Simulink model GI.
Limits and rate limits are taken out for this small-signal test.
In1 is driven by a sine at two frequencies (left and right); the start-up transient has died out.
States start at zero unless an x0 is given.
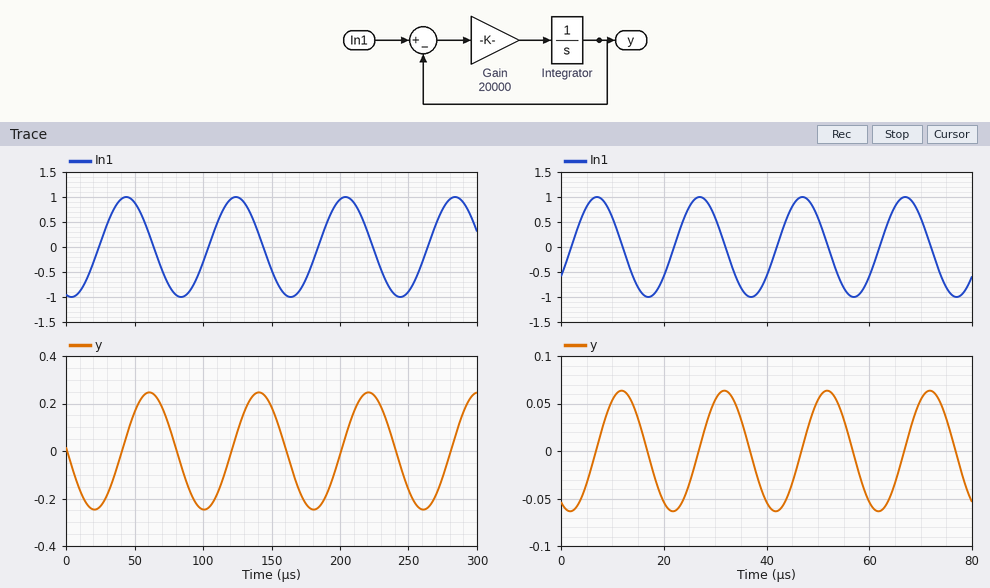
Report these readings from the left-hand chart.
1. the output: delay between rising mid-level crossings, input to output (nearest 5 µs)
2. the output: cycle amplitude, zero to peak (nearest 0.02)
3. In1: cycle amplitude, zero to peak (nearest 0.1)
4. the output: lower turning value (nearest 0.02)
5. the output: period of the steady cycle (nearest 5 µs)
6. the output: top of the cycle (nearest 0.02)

15 µs
0.24
1.0
-0.24
80 µs
0.24
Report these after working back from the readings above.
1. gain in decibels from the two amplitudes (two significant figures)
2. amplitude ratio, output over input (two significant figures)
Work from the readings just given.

-12 dB
0.24
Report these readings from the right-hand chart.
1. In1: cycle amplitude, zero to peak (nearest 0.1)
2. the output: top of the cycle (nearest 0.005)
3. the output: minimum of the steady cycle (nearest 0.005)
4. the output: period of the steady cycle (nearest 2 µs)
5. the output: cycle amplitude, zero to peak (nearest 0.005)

1.0
0.065
-0.065
20 µs
0.065
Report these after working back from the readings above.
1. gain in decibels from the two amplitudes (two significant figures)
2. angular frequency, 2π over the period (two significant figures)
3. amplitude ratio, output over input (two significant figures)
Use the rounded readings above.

-24 dB
0.31 rad/µs
0.065
